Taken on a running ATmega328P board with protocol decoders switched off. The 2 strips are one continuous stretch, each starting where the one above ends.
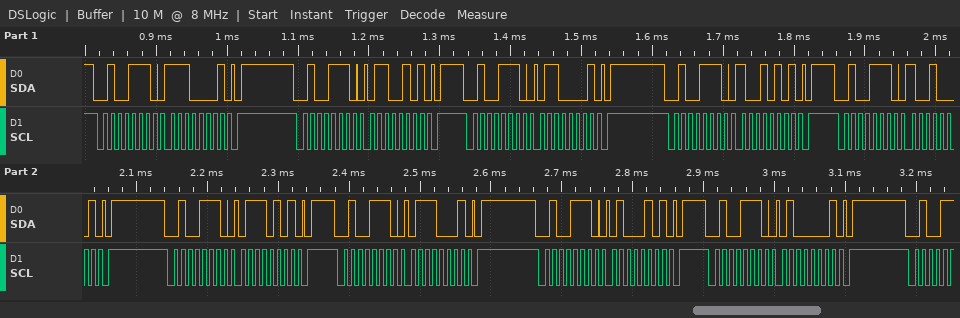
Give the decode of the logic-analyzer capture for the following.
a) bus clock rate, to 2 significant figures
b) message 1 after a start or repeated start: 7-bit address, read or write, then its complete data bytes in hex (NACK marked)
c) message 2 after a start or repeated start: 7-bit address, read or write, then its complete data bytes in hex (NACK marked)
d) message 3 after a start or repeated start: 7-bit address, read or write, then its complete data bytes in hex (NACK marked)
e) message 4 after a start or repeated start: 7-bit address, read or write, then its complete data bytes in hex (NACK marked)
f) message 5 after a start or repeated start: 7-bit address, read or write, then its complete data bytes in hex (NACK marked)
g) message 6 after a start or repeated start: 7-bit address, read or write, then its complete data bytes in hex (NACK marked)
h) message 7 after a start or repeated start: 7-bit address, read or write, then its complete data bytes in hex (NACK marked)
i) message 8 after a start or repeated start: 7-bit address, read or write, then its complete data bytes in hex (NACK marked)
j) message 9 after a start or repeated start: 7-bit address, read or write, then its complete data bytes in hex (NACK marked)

100 kHz
0x27 write: E1
0x27 write: 65
0x27 write: 61
0x27 write: 95
0x27 write: 91
0x27 write: 75
0x27 write: 71
0x27 write: 45
0x27 write: 41
